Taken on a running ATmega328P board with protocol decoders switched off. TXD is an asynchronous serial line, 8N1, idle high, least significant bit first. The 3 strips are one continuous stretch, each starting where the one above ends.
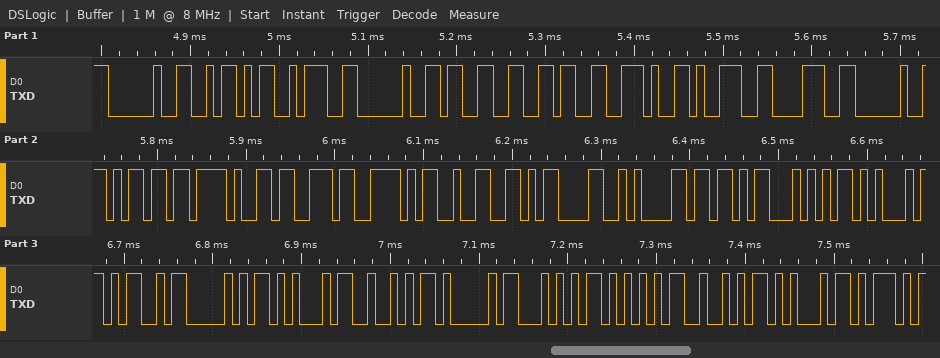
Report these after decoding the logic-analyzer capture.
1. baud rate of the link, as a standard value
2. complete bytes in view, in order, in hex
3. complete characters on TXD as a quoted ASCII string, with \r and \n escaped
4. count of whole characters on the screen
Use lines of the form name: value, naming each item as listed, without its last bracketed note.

baud rate of the link, as a standard value: 115200 baud
complete bytes in view, in order, in hex: 20 5A 3A 20 33 36 2E 39 38 20 6D 2F 73 5E 32 0D 0A 5B 54 45 4D 50 45 52 41 54 55 52 45 5D
complete characters on TXD as a quoted ASCII string, with \r and \n escaped: " Z: 36.98 m/s^2\r\n[TEMPERATURE]"
count of whole characters on the screen: 30
